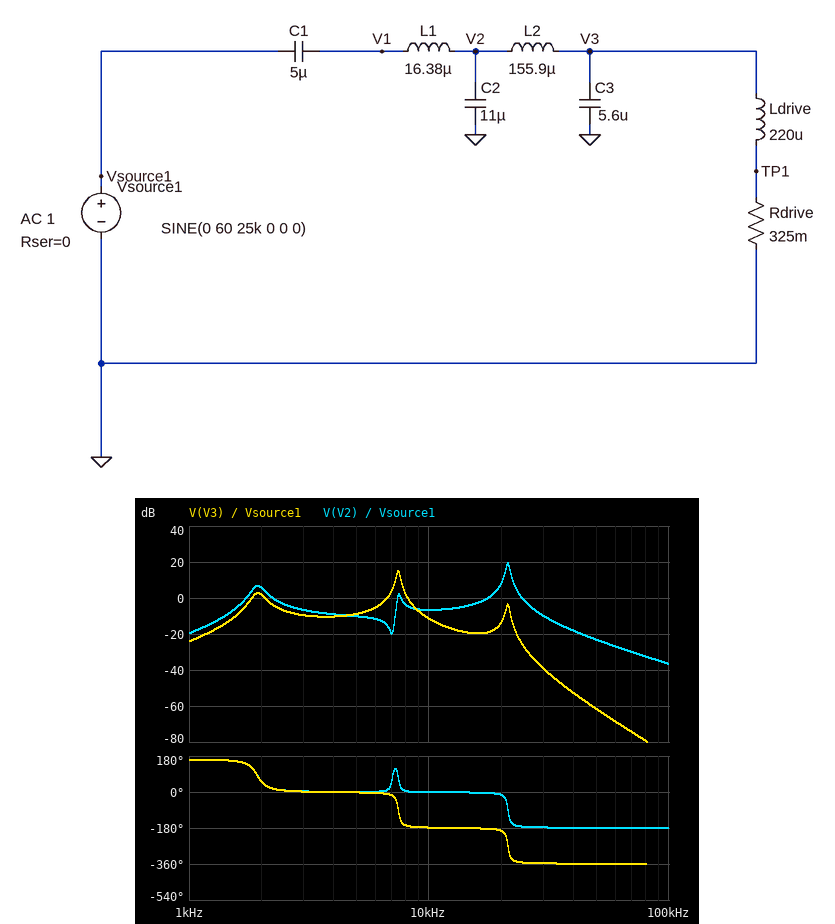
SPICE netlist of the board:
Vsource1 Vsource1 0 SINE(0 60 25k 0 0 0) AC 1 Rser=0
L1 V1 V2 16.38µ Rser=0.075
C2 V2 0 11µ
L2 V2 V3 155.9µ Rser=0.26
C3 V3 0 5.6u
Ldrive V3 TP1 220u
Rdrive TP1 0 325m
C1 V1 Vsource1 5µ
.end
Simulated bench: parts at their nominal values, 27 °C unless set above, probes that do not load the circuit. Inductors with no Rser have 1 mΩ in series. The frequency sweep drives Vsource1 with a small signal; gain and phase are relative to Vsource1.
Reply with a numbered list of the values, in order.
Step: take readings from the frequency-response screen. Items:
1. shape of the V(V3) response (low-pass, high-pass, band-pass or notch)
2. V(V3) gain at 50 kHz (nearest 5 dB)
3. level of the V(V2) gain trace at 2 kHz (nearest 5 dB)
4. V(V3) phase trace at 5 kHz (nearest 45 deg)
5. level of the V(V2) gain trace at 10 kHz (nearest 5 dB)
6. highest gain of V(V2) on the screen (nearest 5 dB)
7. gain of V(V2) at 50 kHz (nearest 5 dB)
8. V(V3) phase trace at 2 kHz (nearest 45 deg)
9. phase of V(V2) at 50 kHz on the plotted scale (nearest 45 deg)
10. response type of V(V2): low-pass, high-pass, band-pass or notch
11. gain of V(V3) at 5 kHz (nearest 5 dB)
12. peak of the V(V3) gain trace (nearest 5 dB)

1. band-pass
2. -60 dB
3. 5 dB
4. 0 deg
5. -5 dB
6. 20 dB
7. -25 dB
8. 45 deg
9. -180 deg
10. band-pass
11. -10 dB
12. 15 dB
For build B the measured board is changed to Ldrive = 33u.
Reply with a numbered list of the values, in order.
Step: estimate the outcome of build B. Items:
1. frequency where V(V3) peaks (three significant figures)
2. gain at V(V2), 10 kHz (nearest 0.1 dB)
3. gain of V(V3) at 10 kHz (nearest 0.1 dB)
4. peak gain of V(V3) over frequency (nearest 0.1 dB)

1. 21.3 kHz
2. -7.5 dB
3. -14.7 dB
4. -0.6 dB
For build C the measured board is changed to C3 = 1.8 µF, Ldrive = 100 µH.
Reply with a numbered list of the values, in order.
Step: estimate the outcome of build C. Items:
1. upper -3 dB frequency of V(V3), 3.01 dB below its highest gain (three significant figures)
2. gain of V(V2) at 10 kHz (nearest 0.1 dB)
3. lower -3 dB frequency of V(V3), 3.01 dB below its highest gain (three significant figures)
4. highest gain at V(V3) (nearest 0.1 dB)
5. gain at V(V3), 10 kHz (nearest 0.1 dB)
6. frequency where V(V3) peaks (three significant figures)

1. 15.5 kHz
2. -7.7 dB
3. 15.1 kHz
4. 19.1 dB
5. -10.9 dB
6. 15.3 kHz
